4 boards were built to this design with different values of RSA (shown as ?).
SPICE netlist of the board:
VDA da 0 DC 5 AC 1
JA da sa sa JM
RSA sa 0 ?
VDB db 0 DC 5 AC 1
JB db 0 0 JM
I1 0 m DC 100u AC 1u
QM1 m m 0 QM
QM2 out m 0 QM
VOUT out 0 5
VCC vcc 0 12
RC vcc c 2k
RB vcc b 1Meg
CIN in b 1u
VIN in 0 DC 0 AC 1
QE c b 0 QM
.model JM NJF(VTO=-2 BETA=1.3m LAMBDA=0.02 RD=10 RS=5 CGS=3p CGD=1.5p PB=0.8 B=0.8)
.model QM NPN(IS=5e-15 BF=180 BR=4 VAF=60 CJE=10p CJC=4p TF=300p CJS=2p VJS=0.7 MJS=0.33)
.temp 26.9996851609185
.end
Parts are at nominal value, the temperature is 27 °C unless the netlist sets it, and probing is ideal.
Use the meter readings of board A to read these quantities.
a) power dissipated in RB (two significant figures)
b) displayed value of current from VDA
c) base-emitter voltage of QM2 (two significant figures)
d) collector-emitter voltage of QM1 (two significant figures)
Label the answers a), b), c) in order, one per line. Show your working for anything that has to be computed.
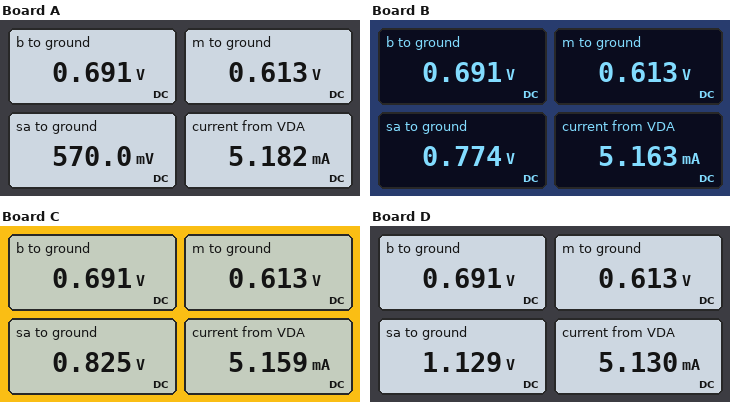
a) (12 V - 691 mV)^2 / 1 MΩ = 130 µW
b) 5.182 mA
c) 613 mV = 610 mV
d) 613 mV = 610 mV
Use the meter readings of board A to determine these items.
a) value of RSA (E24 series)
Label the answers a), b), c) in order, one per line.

a) 110 Ω
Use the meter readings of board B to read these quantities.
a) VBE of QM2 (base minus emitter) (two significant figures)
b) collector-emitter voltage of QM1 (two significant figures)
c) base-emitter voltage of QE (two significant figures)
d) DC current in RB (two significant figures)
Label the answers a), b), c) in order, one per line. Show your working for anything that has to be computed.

a) 613 mV = 610 mV
b) 613 mV = 610 mV
c) 691 mV = 690 mV
d) (12 V - 691 mV) / 1 MΩ = 11 µA
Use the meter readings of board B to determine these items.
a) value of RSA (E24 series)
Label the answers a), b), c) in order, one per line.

a) 150 Ω
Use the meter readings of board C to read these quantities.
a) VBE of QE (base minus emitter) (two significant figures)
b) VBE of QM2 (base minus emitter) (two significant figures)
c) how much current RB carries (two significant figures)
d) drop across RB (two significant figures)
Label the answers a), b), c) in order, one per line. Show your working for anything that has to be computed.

a) 691 mV = 690 mV
b) 613 mV = 610 mV
c) (12 V - 691 mV) / 1 MΩ = 11 µA
d) 12 V - 691 mV = 11 V
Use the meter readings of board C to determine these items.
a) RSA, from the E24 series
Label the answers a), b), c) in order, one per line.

a) 160 Ω
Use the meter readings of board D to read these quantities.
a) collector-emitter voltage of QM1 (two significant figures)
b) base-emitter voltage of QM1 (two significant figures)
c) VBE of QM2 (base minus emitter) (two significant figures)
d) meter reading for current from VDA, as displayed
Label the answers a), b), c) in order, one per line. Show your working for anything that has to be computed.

a) 613 mV = 610 mV
b) 613 mV = 610 mV
c) 613 mV = 610 mV
d) 5.130 mA
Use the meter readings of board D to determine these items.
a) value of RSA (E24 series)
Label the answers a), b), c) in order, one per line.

a) 220 Ω
